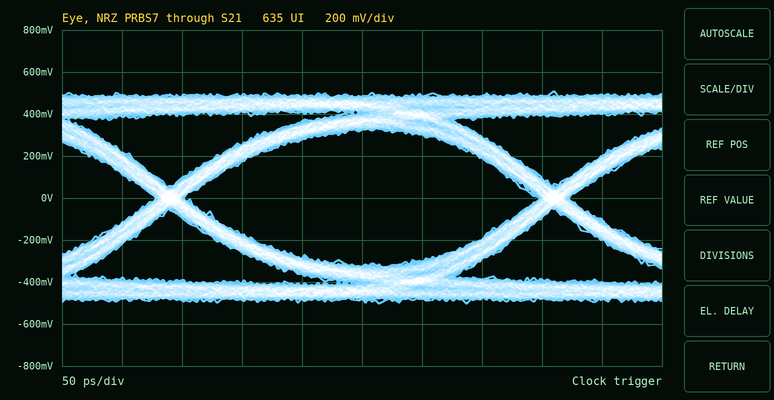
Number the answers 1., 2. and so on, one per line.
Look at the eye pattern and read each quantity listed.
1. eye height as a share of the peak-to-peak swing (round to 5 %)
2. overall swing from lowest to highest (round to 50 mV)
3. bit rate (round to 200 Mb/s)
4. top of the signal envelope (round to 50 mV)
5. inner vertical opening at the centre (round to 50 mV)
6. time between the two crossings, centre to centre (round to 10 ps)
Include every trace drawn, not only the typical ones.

1. 65 %
2. 1.00 V
3. 3.2 Gb/s
4. 500 mV
5. 650 mV
6. 320 ps
